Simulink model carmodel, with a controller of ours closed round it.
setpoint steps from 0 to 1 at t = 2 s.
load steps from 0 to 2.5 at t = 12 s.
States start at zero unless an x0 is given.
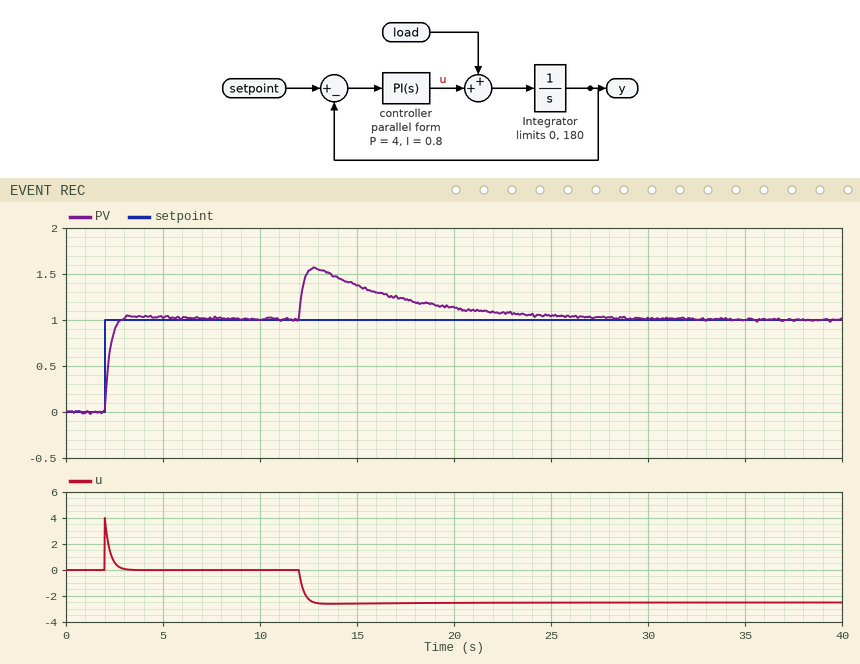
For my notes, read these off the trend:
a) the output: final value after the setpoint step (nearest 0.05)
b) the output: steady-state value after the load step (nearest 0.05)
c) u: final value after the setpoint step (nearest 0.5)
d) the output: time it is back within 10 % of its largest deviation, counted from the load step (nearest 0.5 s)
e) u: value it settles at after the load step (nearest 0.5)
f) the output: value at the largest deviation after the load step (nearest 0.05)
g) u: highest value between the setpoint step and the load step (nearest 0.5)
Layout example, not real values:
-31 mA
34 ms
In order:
1.00
1.00
0.0
12.0 s
-2.5
1.55
4.0
